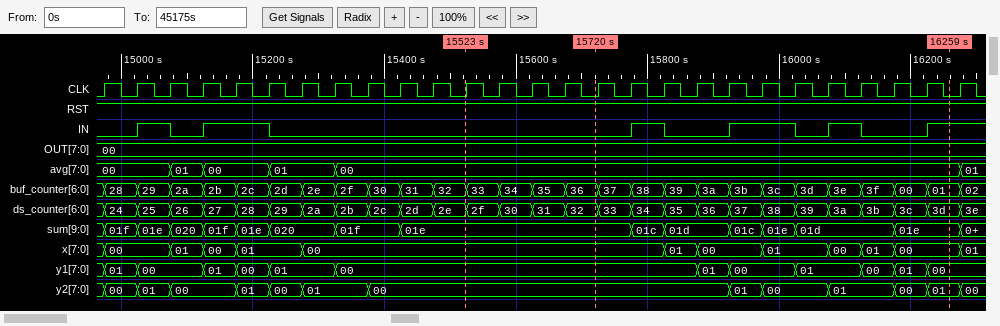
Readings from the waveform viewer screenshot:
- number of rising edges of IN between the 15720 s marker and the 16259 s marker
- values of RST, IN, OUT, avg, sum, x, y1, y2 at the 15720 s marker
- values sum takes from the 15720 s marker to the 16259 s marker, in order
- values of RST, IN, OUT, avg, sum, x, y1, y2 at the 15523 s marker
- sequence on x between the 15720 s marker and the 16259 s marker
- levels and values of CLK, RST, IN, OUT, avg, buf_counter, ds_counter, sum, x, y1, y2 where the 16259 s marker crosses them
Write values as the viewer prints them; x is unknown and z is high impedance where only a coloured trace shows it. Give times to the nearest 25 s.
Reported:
4
RST=1, IN=0, OUT=00, avg=00, sum=01e, x=00, y1=00, y2=00
01e, 01c, 01d, 01c, 01e, 01d, 01e
RST=1, IN=0, OUT=00, avg=00, sum=01e, x=00, y1=00, y2=00
00, 01, 00, 01, 00, 01, 00
CLK=0, RST=1, IN=1, OUT=00, avg=00, buf_counter=01, ds_counter=3d, sum=01e, x=00, y1=00, y2=01
